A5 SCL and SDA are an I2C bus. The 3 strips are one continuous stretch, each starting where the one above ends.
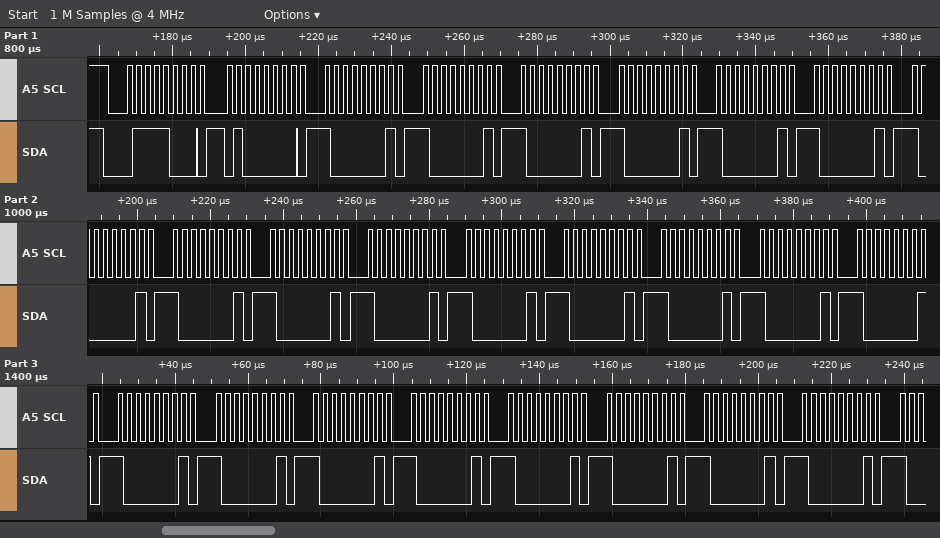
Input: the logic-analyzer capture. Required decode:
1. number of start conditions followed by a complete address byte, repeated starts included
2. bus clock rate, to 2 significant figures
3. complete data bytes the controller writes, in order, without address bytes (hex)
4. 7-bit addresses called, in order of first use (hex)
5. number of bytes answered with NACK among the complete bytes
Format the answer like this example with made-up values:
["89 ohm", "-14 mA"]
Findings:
["1", "400 kHz", "40 81 81 81 81 81 81 81 81 81 81 81 81 81 81 81 81 81 81 81 81 81 81 81", "0x3C", "0"]
